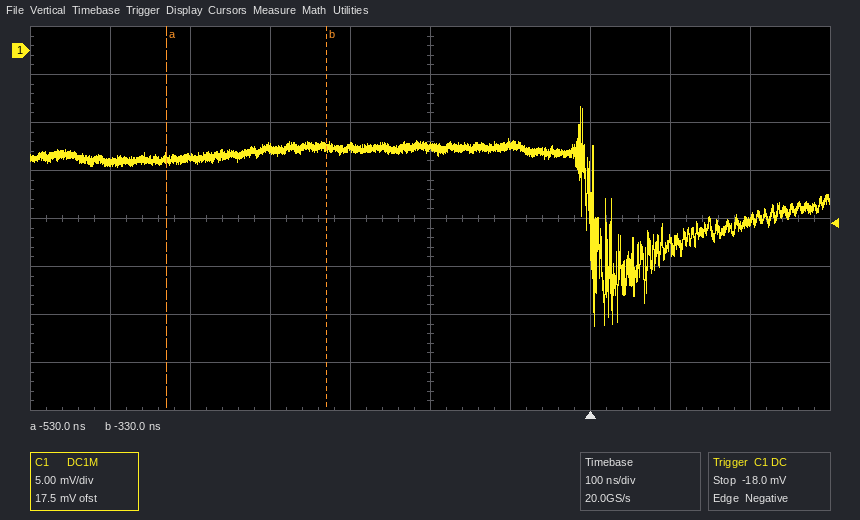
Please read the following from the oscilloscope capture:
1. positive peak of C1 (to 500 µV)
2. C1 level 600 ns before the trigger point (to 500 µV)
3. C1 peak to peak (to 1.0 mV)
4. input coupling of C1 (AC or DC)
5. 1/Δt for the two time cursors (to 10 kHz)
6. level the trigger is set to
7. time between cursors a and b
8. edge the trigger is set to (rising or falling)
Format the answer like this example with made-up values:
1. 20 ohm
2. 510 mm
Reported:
1. -6.0 mV
2. -11.5 mV
3. 23.0 mV
4. DC
5. 5.00 MHz
6. -18.0 mV
7. 200 ns
8. falling
